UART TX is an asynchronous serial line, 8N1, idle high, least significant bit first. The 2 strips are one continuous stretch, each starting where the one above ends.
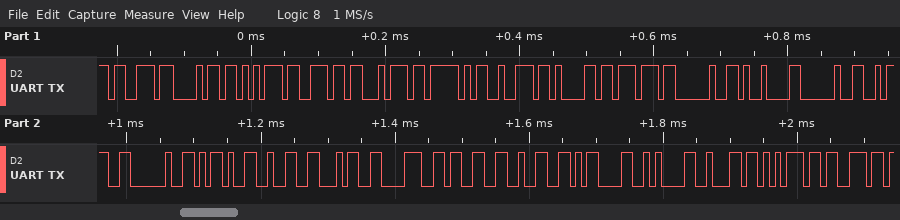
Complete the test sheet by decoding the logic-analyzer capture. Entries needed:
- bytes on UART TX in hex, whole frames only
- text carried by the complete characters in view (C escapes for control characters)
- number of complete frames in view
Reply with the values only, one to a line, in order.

0x73 0x68 0x75 0x6E 0x74 0x5F 0x72 0x61 0x77 0x20 0x09 0x20 0x3A 0x20 0x2D 0x32 0x34 0x38 0x33 0x32 0x0D 0x0A 0x62 0x75 0x73
"shunt_raw \t : -24832\r\nbus"
25
